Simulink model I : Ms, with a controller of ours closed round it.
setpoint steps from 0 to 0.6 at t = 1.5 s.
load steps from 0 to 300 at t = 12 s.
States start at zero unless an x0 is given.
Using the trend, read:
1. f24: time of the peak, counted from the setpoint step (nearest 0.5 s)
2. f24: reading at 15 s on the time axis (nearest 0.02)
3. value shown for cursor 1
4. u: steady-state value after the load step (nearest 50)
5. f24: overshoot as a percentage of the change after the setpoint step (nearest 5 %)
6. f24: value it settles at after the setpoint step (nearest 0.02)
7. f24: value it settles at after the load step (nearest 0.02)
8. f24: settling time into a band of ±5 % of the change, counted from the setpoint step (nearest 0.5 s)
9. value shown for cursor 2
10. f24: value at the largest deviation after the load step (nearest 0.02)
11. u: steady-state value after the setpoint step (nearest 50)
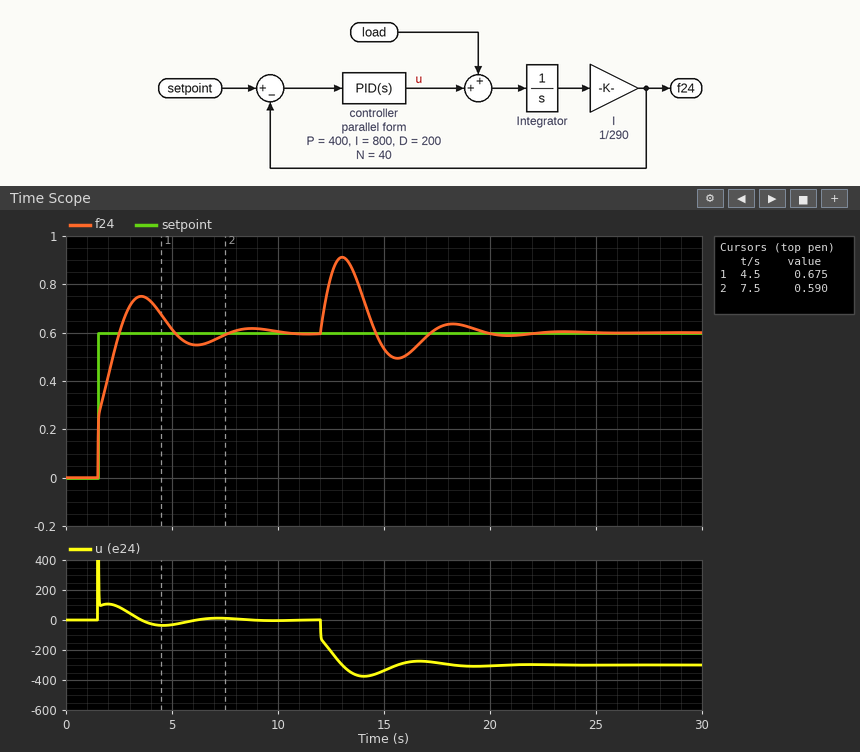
2.0 s
0.54
0.675
-300
25 %
0.60
0.60
5.5 s
0.590
0.92
0
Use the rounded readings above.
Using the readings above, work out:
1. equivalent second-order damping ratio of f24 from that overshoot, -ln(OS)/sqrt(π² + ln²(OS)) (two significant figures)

0.40
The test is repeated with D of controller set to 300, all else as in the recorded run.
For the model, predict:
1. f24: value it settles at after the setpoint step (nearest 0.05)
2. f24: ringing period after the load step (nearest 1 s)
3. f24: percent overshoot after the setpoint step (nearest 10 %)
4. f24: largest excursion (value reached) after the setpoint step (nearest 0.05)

0.60
6 s
20 %
0.75
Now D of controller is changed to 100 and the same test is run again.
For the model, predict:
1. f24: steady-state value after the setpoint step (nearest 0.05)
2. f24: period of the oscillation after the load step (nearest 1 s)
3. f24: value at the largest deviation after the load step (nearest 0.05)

0.60
5 s
0.95
